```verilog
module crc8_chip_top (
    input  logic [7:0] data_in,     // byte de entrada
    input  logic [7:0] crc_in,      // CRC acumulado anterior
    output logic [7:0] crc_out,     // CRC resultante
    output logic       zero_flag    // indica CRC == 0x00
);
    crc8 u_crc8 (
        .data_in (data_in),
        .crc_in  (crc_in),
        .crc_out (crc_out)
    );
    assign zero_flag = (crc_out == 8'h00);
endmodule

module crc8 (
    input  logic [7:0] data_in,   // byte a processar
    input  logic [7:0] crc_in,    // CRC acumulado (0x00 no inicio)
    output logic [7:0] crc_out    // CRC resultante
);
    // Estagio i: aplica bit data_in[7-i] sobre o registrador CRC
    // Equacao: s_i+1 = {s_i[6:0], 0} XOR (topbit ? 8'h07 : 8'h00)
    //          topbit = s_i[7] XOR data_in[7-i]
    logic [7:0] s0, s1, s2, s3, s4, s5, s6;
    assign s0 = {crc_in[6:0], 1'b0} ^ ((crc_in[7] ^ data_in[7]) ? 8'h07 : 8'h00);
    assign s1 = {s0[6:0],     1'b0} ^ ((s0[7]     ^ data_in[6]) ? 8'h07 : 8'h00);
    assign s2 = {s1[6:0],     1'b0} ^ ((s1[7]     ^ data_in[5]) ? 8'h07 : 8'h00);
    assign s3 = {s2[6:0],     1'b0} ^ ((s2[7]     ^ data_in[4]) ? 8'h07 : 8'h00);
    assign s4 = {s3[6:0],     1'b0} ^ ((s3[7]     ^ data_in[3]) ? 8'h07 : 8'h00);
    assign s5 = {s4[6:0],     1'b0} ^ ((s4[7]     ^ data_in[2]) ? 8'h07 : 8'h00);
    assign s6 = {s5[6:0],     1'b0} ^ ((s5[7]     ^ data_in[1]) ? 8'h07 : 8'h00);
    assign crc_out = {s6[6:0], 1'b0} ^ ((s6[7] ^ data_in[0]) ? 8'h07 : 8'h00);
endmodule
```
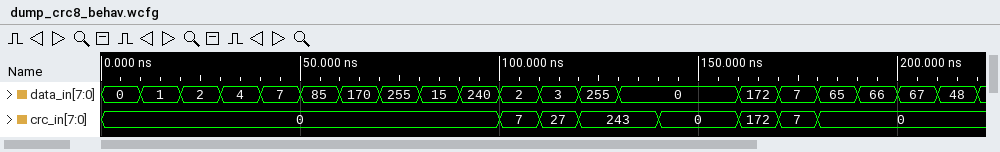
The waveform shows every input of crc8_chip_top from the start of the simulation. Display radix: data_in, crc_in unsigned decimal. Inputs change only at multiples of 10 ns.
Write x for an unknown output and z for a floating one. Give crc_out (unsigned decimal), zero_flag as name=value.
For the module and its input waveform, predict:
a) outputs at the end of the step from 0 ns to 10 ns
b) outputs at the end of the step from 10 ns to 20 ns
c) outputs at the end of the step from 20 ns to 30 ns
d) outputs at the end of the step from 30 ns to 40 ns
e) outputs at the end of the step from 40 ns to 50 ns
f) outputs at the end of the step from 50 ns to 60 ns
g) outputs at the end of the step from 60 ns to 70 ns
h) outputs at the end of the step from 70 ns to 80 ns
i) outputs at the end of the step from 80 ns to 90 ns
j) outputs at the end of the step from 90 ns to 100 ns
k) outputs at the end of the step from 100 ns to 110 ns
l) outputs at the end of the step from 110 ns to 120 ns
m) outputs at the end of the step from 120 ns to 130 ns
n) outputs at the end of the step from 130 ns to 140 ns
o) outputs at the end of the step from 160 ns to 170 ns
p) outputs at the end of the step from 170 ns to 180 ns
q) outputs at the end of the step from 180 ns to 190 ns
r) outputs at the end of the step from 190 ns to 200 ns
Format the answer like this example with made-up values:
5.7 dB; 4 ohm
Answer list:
crc_out=0, zero_flag=1; crc_out=7, zero_flag=0; crc_out=14, zero_flag=0; crc_out=28, zero_flag=0; crc_out=21, zero_flag=0; crc_out=172, zero_flag=0; crc_out=95, zero_flag=0; crc_out=243, zero_flag=0; crc_out=45, zero_flag=0; crc_out=222, zero_flag=0; crc_out=27, zero_flag=0; crc_out=72, zero_flag=0; crc_out=36, zero_flag=0; crc_out=215, zero_flag=0; crc_out=0, zero_flag=1; crc_out=0, zero_flag=1; crc_out=192, zero_flag=0; crc_out=201, zero_flag=0
